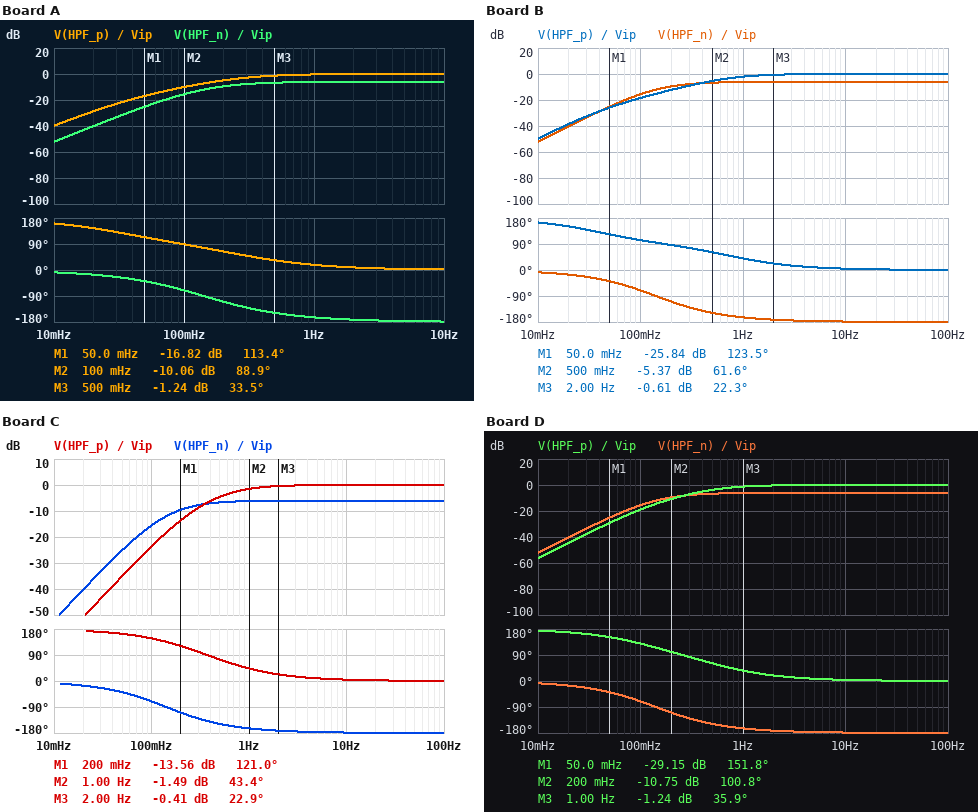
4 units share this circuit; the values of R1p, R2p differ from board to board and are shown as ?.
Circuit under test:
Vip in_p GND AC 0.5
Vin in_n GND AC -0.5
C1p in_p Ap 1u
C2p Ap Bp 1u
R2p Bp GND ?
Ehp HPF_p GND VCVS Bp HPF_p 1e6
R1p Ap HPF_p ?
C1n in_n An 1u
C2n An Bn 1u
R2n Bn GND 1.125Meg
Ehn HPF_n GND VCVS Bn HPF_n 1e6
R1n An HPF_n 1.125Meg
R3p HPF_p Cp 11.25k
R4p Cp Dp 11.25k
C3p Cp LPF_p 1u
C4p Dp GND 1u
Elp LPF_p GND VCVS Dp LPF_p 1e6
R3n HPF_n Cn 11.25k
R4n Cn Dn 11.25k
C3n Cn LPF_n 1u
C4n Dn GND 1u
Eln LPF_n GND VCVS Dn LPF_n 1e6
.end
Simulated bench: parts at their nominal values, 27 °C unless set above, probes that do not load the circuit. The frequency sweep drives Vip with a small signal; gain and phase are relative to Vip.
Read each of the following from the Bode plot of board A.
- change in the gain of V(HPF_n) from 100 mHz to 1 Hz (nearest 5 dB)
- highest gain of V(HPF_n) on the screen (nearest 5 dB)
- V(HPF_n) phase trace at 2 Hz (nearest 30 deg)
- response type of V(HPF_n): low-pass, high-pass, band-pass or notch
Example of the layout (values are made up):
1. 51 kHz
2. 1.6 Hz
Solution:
1. 10 dB
2. -5 dB
3. -180 deg
4. high-pass
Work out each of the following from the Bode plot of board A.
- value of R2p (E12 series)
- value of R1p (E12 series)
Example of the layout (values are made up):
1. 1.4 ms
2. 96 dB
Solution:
1. 1 MΩ
2. 2.7 MΩ
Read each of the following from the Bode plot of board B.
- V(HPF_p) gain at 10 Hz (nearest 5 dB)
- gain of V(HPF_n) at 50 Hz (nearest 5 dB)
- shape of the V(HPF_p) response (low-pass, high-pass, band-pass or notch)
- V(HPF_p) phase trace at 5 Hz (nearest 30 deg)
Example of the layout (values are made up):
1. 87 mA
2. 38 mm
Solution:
1. 0 dB
2. -5 dB
3. high-pass
4. 0 deg
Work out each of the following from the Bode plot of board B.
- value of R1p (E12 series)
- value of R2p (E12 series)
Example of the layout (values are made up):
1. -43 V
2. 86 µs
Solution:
1. 2.2 MΩ
2. 390 kΩ
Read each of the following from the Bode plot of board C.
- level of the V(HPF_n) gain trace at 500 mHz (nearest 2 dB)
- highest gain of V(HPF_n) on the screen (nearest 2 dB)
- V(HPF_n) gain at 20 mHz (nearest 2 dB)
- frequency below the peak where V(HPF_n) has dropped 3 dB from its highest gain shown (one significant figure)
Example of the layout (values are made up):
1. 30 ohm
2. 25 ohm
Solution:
1. -6 dB
2. -6 dB
3. -40 dB
4. 200 mHz
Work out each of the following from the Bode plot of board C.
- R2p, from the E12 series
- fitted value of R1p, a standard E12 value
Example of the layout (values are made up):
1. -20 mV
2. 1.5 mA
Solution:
1. 390 kΩ
2. 470 kΩ
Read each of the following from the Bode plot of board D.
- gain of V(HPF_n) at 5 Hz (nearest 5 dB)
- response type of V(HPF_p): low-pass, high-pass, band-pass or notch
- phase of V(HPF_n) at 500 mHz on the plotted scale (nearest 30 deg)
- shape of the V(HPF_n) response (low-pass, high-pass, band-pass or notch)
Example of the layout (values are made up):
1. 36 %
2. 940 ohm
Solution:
1. -5 dB
2. high-pass
3. -150 deg
4. high-pass
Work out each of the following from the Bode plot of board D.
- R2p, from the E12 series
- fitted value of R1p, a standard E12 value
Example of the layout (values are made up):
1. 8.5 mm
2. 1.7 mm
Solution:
1. 470 kΩ
2. 820 kΩ
